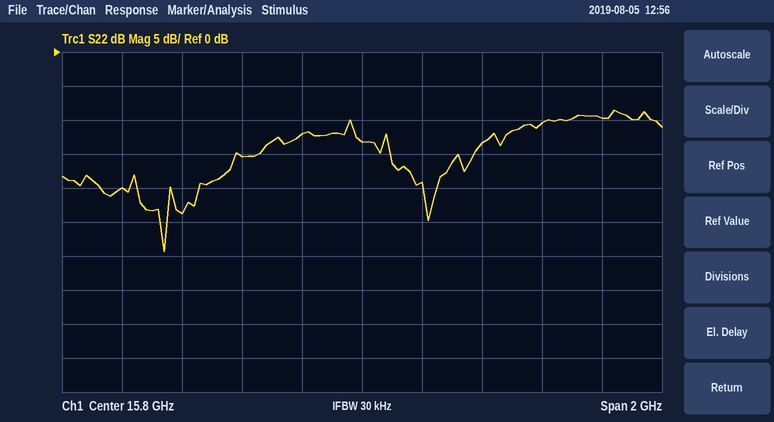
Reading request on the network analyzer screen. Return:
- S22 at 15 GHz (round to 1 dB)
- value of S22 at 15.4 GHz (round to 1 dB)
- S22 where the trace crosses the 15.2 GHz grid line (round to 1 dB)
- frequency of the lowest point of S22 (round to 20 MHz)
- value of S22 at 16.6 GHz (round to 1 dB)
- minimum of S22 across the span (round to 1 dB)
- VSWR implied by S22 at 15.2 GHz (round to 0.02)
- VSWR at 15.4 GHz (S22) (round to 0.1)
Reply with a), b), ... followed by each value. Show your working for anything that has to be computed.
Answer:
a) -20 dB
b) -15 dB
c) -24 dB
d) 15.14 GHz
e) -10 dB
f) -29 dB
g) |Γ| = 10^(-24/20) = 0.0631; VSWR = (1 + 0.0631)/(1 − 0.0631) ≈ 1.13, so 1.14 to the nearest 0.02
h) |Γ| = 10^(-15/20) = 0.1778; VSWR = (1 + 0.1778)/(1 − 0.1778) ≈ 1.4
